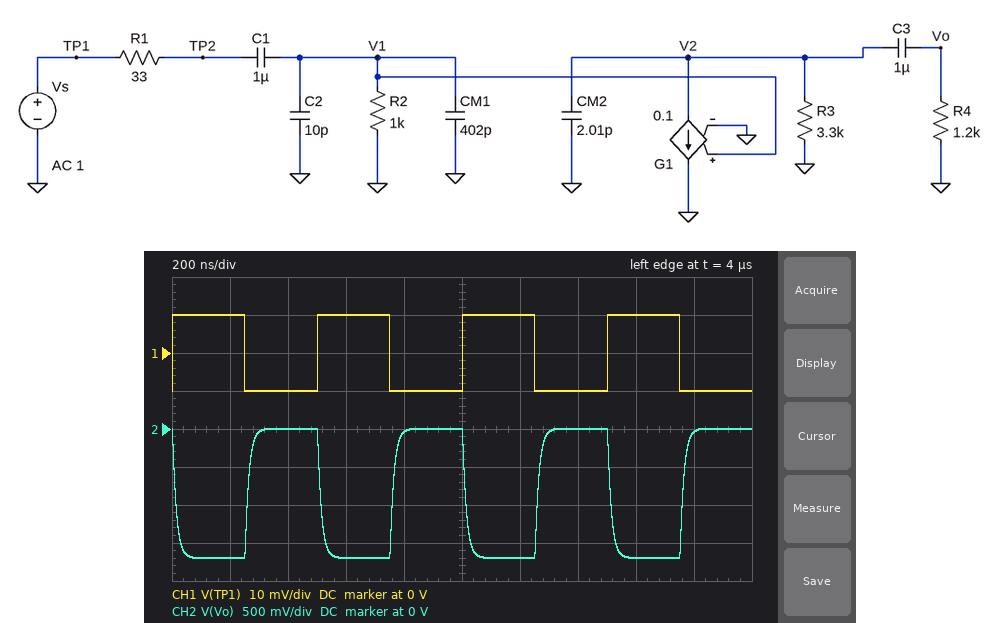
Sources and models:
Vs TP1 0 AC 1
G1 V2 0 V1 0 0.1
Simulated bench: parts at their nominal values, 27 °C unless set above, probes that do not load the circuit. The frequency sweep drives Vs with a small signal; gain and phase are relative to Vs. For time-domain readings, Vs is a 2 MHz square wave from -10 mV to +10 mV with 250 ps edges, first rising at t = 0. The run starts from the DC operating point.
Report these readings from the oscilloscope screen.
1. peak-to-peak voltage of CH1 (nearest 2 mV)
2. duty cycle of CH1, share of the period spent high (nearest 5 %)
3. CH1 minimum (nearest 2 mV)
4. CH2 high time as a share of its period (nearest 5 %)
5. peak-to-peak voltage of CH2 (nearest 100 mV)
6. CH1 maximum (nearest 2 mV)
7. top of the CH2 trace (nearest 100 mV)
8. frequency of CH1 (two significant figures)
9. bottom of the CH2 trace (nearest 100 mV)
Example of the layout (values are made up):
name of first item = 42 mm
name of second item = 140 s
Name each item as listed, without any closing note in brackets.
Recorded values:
peak-to-peak voltage of CH1 = 20 mV
duty cycle of CH1, share of the period spent high = 50 %
CH1 minimum = -10 mV
CH2 high time as a share of its period = 50 %
peak-to-peak voltage of CH2 = 1.7 V
CH1 maximum = 10 mV
top of the CH2 trace = 0 V
frequency of CH1 = 2.0 MHz
bottom of the CH2 trace = -1.7 V
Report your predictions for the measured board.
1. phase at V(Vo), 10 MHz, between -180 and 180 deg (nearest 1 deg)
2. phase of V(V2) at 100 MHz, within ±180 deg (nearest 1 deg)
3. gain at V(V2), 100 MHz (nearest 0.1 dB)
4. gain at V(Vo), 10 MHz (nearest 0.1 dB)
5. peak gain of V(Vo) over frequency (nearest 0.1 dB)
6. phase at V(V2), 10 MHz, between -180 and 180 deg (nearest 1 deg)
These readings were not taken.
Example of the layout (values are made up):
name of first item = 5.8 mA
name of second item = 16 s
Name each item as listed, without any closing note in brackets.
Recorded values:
phase at V(Vo), 10 MHz, between -180 and 180 deg = 134 deg
phase of V(V2) at 100 MHz, within ±180 deg = 49 deg
gain at V(V2), 100 MHz = 16.7 dB
gain at V(Vo), 10 MHz = 36.3 dB
peak gain of V(Vo) over frequency = 38.6 dB
phase at V(V2), 10 MHz, between -180 and 180 deg = 134 deg
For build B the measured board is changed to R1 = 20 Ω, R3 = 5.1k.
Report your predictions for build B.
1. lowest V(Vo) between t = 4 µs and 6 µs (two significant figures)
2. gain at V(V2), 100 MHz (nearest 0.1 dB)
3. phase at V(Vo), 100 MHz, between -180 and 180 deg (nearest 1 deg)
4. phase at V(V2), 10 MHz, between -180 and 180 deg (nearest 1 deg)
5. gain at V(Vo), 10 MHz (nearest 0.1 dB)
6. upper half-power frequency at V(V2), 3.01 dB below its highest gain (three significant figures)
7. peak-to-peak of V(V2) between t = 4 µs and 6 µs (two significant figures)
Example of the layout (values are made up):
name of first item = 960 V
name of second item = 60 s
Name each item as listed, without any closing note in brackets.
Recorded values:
lowest V(Vo) between t = 4 µs and 6 µs = -1.9 V
gain at V(V2), 100 MHz = 21.3 dB
phase at V(Vo), 100 MHz, between -180 and 180 deg = 50 deg
phase at V(V2), 10 MHz, between -180 and 180 deg = 146 deg
gain at V(Vo), 10 MHz = 38.5 dB
upper half-power frequency at V(V2), 3.01 dB below its highest gain = 18.7 MHz
peak-to-peak of V(V2) between t = 4 µs and 6 µs = 1.9 V
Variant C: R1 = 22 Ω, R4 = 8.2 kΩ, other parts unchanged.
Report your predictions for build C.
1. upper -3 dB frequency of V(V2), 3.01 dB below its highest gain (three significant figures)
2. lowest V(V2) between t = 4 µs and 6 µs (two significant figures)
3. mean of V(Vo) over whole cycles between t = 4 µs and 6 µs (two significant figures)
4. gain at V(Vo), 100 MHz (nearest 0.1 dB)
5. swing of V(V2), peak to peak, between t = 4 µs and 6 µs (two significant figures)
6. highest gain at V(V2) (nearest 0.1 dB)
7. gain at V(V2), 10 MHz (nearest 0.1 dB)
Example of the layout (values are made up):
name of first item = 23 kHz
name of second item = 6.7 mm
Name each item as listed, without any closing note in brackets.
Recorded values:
upper -3 dB frequency of V(V2), 3.01 dB below its highest gain = 14.8 MHz
lowest V(V2) between t = 4 µs and 6 µs = -4.6 V
mean of V(Vo) over whole cycles between t = 4 µs and 6 µs = -2.3 V
gain at V(Vo), 100 MHz = 22.3 dB
swing of V(V2), peak to peak, between t = 4 µs and 6 µs = 4.6 V
highest gain at V(V2) = 47.2 dB
gain at V(V2), 10 MHz = 45.7 dB
